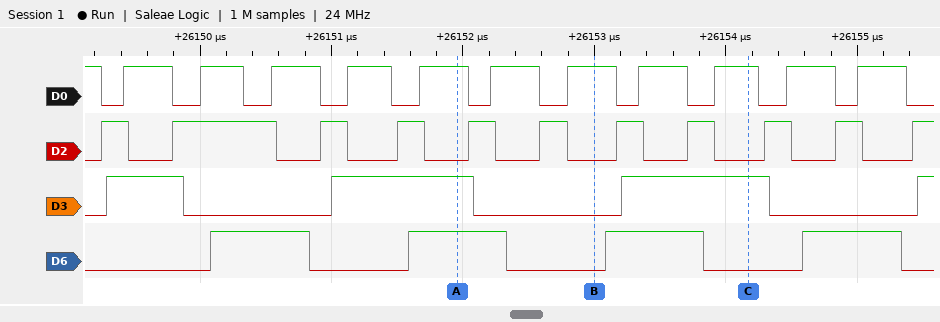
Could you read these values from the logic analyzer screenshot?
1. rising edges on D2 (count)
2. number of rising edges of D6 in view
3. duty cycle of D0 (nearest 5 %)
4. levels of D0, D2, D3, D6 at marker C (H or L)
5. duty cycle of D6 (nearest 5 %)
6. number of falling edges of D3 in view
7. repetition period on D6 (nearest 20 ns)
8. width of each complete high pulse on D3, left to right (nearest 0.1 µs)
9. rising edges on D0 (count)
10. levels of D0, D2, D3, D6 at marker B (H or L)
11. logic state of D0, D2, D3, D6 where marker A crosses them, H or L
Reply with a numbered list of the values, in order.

1. 11
2. 4
3. 65 %
4. D0=H, D2=L, D3=H, D6=L
5. 50 %
6. 3
7. 1500 ns
8. 0.6 µs, 1.1 µs, 1.1 µs
9. 11
10. D0=H, D2=L, D3=L, D6=L
11. D0=H, D2=L, D3=H, D6=H
